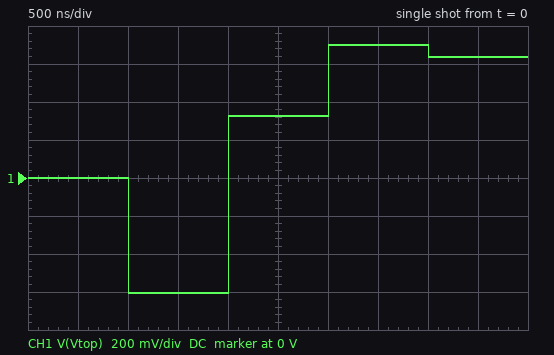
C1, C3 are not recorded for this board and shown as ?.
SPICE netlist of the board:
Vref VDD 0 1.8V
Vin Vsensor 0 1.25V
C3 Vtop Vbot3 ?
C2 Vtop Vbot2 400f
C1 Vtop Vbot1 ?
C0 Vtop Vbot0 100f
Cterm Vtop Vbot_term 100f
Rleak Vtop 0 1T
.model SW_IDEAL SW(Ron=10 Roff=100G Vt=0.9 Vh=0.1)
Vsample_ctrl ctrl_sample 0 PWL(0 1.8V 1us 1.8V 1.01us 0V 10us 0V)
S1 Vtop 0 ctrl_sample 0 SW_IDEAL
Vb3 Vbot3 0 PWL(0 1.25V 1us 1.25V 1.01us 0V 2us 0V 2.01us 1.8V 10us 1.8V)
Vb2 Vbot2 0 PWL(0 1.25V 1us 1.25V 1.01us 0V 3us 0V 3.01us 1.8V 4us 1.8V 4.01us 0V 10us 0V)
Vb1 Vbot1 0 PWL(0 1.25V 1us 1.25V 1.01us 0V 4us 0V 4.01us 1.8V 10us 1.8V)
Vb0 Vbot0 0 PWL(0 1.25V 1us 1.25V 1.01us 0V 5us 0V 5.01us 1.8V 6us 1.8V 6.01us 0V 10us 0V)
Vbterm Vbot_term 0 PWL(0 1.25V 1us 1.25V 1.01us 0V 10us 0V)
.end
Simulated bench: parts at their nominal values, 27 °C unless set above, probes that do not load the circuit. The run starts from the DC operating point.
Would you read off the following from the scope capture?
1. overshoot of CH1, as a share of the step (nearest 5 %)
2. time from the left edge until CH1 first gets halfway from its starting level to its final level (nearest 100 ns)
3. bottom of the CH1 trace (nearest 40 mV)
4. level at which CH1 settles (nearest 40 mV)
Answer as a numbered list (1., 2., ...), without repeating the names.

1. 10 %
2. 2.0 µs
3. -600 mV
4. 640 mV
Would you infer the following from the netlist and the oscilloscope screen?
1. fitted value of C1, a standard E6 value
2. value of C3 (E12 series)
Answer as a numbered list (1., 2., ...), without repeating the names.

1. 330 fF
2. 1 pF
